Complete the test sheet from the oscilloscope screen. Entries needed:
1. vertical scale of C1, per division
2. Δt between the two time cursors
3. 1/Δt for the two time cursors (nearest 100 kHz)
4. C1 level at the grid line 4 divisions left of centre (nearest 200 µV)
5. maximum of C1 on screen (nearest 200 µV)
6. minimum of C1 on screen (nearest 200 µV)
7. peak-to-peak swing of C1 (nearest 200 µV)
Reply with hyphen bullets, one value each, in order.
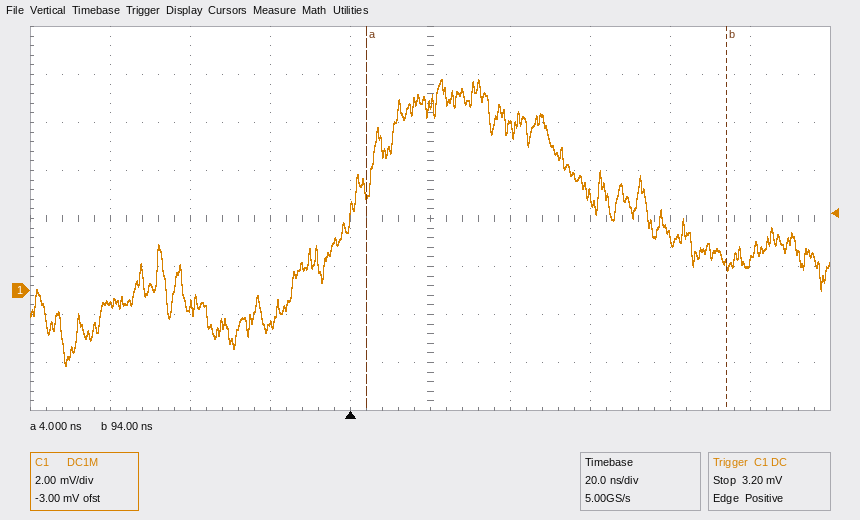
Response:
- 2 mV
- 90 ns
- 11.1 MHz
- -600 µV
- 8.8 mV
- -3.2 mV
- 12.0 mV
